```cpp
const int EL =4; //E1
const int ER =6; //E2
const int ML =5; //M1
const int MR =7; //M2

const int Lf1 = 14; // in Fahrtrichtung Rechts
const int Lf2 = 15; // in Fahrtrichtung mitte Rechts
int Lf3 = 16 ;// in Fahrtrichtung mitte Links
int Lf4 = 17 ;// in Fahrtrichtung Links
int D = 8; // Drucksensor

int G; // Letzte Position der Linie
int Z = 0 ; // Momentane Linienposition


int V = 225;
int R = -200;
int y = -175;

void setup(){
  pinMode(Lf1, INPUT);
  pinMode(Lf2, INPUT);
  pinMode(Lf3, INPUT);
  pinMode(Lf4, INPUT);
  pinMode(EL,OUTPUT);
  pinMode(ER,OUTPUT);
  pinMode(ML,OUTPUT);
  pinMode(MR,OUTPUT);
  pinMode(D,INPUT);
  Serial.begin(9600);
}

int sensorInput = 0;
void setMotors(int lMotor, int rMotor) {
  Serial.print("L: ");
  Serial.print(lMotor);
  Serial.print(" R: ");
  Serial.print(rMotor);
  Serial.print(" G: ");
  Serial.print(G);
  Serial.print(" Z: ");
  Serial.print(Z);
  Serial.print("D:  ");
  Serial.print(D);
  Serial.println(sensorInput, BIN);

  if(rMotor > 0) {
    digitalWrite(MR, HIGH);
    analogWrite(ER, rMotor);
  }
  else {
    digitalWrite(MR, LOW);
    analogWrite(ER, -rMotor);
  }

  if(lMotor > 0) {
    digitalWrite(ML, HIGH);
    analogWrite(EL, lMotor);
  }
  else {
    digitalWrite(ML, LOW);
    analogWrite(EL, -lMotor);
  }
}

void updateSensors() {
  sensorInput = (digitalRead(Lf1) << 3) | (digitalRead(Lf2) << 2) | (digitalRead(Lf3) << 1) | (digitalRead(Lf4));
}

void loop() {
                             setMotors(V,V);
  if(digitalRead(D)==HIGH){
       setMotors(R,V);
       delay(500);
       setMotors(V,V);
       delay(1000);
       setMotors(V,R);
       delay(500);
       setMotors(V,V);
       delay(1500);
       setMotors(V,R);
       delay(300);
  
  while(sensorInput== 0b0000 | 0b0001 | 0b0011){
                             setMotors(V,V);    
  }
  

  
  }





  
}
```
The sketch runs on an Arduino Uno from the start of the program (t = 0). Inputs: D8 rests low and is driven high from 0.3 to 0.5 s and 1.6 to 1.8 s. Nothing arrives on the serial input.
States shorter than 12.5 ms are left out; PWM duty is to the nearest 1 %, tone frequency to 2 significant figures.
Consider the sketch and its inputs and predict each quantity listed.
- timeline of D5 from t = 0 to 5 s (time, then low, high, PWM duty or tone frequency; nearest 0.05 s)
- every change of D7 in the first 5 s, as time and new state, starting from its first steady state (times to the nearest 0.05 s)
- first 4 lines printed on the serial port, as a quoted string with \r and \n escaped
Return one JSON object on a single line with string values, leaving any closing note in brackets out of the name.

{"timeline of D5 from t = 0 to 5 s": "0 s high; 0.35 s low; 0.85 s high", "every change of D7 in the first 5 s, as time and new state, starting from its first steady state": "0 s high; 1.85 s low; 2.35 s high; 3.85 s low; 4.15 s high", "first 4 lines printed on the serial port, as a quoted string with \\r and \\n escaped": "\"L: 225 R: 225 G: 0 Z: 0D:  80\\r\\nL: 225 R: 225 G: 0 Z: 0D:  80\\r\\nL: 225 R: 225 G: 0 Z: 0D:  80\\r\\nL: 225 R: 225 G: 0 Z: 0D:  80\\r\\n\""}
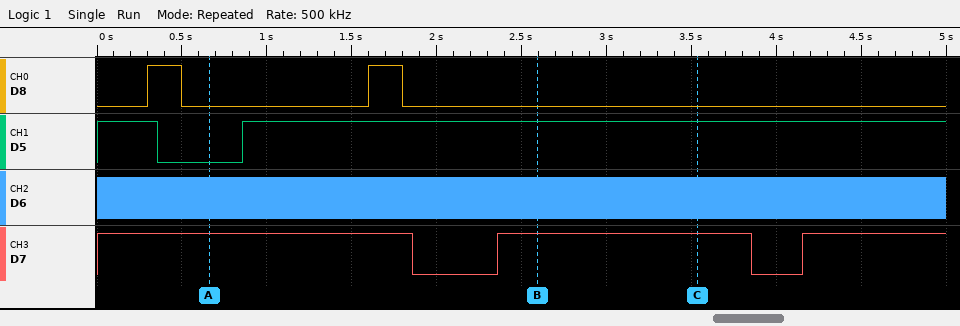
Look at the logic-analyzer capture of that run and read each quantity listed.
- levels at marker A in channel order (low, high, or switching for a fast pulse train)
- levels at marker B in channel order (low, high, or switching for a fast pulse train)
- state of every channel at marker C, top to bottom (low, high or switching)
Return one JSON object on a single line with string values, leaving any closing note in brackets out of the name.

{"levels at marker A in channel order": "D8 low, D5 low, D6 switching, D7 high", "levels at marker B in channel order": "D8 low, D5 high, D6 switching, D7 high", "state of every channel at marker C, top to bottom": "D8 low, D5 high, D6 switching, D7 high"}
